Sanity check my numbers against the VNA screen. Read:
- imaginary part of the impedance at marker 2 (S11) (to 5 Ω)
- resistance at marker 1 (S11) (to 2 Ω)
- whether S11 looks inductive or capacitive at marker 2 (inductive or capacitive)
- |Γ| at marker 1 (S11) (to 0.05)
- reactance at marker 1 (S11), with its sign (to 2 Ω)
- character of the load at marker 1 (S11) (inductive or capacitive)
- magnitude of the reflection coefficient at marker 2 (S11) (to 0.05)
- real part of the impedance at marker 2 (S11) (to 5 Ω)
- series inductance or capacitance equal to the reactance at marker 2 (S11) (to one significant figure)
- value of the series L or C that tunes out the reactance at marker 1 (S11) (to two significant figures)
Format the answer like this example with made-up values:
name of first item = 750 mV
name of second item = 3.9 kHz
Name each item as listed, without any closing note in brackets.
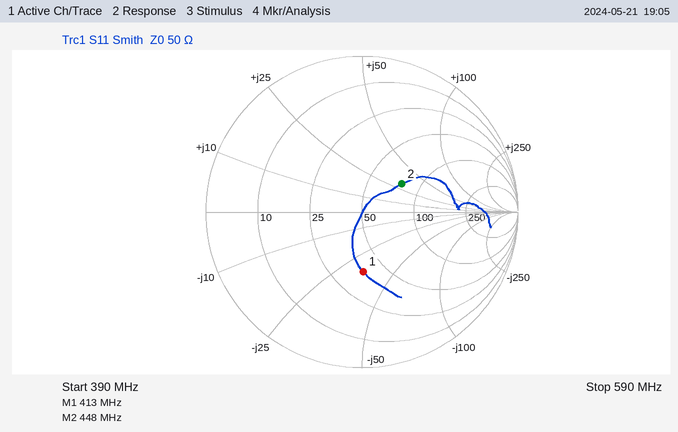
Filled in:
imaginary part of the impedance at marker 2 (S11) = +30 Ω
resistance at marker 1 (S11) = 38 Ω
whether S11 looks inductive or capacitive at marker 2 = inductive
|Γ| at marker 1 (S11) = 0.40
reactance at marker 1 (S11), with its sign = -34 Ω
character of the load at marker 1 (S11) = capacitive
magnitude of the reflection coefficient at marker 2 (S11) = 0.30
real part of the impedance at marker 2 (S11) = 75 Ω
series inductance or capacitance equal to the reactance at marker 2 (S11) = 10 nH
value of the series L or C that tunes out the reactance at marker 1 (S11) = 13 nH
